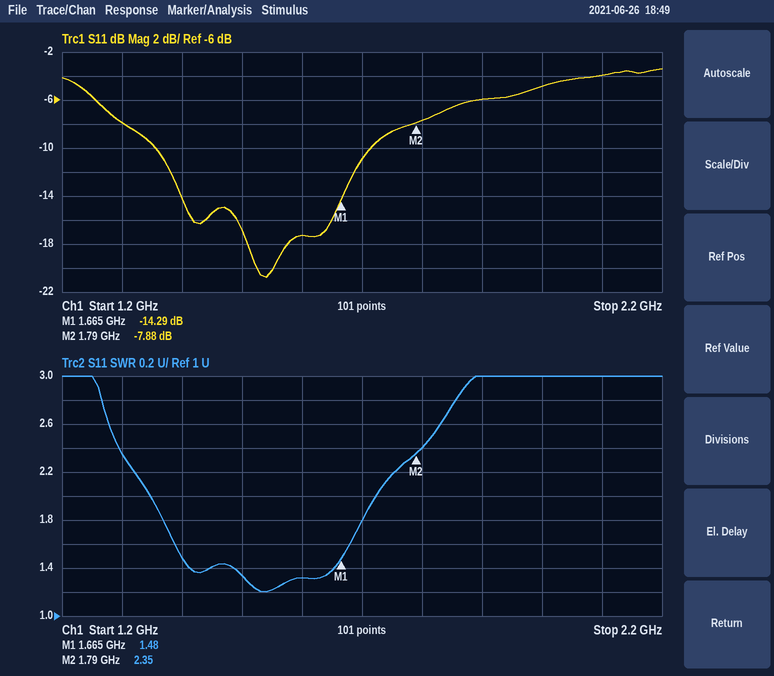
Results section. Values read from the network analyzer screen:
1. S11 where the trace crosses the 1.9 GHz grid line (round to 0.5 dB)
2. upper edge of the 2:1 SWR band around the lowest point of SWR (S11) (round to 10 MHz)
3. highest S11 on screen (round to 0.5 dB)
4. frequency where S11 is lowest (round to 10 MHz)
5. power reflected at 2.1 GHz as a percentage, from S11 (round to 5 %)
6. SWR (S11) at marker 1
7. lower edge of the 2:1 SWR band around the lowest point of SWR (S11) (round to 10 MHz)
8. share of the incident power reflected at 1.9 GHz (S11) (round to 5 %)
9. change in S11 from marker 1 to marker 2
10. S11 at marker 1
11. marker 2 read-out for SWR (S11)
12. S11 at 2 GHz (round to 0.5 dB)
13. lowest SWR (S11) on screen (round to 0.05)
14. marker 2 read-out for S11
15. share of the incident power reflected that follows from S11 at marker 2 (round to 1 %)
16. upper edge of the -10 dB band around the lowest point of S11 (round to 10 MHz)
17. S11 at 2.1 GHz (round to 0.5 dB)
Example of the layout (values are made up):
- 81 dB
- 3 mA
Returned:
- -6.0 dB
- 1.72 GHz
- -3.5 dB
- 1.54 GHz
- 40 %
- 1.48
- 1.35 GHz
- 25 %
- 6.41 dB
- -14.29 dB
- 2.35
- -5.0 dB
- 1.20
- -7.88 dB
- 16 %
- 1.71 GHz
- -4.0 dB
